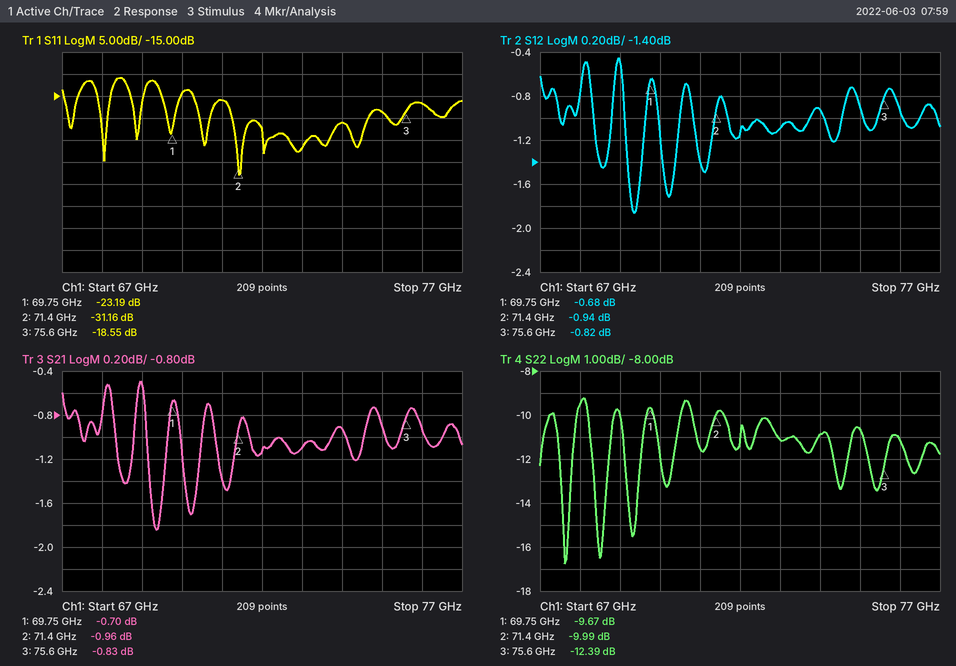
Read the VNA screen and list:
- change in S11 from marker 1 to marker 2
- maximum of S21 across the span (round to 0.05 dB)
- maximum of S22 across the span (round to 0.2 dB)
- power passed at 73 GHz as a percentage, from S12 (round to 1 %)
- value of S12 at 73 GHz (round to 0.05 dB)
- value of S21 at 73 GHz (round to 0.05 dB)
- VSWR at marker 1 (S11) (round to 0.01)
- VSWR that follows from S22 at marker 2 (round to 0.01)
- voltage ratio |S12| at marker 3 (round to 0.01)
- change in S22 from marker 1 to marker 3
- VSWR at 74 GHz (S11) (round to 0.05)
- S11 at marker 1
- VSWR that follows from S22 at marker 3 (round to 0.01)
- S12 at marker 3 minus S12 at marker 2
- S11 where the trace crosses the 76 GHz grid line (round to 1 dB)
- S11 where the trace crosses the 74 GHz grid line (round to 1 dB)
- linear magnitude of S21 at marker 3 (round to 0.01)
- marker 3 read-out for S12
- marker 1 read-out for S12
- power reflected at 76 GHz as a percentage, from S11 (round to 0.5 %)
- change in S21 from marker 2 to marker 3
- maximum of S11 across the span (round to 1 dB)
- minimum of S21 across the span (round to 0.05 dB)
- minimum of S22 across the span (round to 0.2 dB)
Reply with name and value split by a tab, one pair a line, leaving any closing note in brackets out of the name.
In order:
change in S11 from marker 1 to marker 2	-7.97 dB
maximum of S21 across the span	-0.50 dB
maximum of S22 across the span	-9.2 dB
power passed at 73 GHz as a percentage, from S12	78 %
value of S12 at 73 GHz	-1.10 dB
value of S21 at 73 GHz	-1.10 dB
VSWR at marker 1 (S11)	1.15
VSWR that follows from S22 at marker 2	1.93
voltage ratio |S12| at marker 3	0.91
change in S22 from marker 1 to marker 3	-2.72 dB
VSWR at 74 GHz (S11)	1.20
S11 at marker 1	-23.19 dB
VSWR that follows from S22 at marker 3	1.63
S12 at marker 3 minus S12 at marker 2	0.12 dB
S11 where the trace crosses the 76 GHz grid line	-17 dB
S11 where the trace crosses the 74 GHz grid line	-21 dB
linear magnitude of S21 at marker 3	0.91
marker 3 read-out for S12	-0.82 dB
marker 1 read-out for S12	-0.68 dB
power reflected at 76 GHz as a percentage, from S11	2.0 %
change in S21 from marker 2 to marker 3	0.13 dB
maximum of S11 across the span	-11 dB
minimum of S21 across the span	-1.85 dB
minimum of S22 across the span	-16.8 dB
